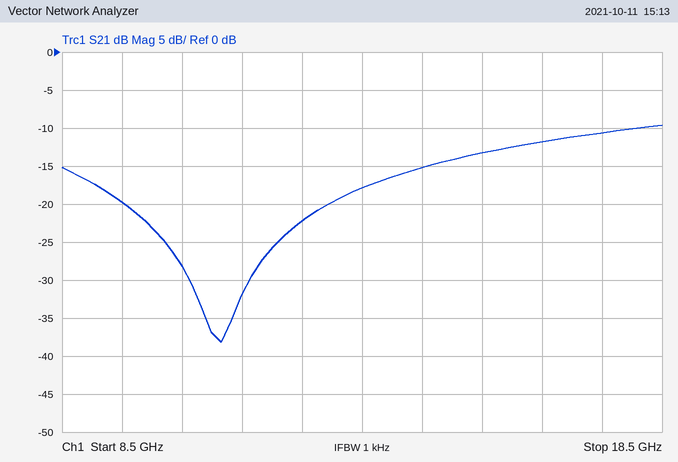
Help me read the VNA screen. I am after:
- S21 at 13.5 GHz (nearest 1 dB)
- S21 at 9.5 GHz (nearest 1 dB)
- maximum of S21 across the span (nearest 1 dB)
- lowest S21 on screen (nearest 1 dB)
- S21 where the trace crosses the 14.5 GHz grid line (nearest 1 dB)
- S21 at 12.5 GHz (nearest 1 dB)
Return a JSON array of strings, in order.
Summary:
["-18 dB", "-20 dB", "-10 dB", "-38 dB", "-15 dB", "-22 dB"]
